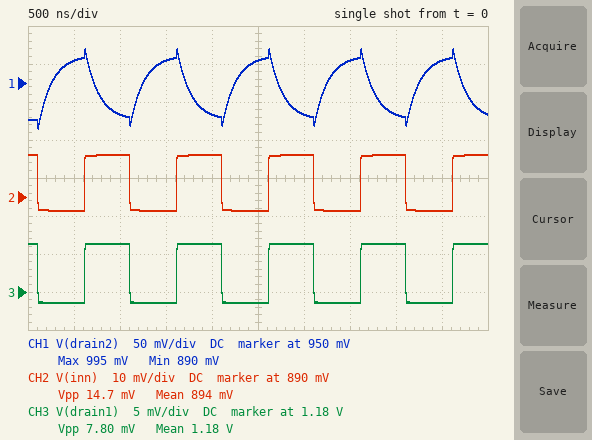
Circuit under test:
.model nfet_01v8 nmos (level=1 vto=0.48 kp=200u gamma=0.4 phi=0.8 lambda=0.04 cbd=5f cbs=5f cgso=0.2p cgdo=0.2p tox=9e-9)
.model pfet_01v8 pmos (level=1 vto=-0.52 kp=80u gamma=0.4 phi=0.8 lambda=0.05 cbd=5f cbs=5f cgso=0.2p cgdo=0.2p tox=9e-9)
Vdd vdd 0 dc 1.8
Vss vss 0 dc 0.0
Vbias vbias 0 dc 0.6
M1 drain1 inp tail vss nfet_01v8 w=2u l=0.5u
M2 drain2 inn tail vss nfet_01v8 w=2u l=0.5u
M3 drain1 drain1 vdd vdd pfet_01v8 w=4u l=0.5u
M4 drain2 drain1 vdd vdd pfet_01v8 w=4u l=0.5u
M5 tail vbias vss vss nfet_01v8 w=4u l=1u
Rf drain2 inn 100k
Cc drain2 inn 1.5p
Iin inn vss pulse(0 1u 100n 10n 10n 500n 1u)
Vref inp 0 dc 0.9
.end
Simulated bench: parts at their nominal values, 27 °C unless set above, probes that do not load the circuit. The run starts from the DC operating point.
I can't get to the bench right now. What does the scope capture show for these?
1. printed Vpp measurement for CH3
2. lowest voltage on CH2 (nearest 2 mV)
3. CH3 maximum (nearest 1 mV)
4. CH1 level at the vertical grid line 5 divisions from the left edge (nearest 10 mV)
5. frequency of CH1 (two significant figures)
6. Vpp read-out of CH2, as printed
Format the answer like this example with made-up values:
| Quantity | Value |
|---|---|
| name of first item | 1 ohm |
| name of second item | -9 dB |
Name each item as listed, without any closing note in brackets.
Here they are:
| Quantity | Value |
|---|---|
| printed Vpp measurement for CH3 | 7.80 mV |
| lowest voltage on CH2 | 886 mV |
| CH3 maximum | 1.186 V |
| CH1 level at the vertical grid line 5 divisions from the left edge | 980 mV |
| frequency of CH1 | 1.0 MHz |
| Vpp read-out of CH2, as printed | 14.7 mV |
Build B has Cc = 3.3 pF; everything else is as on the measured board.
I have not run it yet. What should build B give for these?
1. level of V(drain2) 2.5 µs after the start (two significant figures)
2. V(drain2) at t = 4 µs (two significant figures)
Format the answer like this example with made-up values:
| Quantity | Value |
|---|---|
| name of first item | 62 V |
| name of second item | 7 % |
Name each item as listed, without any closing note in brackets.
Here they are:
| Quantity | Value |
|---|---|
| level of V(drain2) 2.5 µs after the start | 960 mV |
| V(drain2) at t = 4 µs | 930 mV |
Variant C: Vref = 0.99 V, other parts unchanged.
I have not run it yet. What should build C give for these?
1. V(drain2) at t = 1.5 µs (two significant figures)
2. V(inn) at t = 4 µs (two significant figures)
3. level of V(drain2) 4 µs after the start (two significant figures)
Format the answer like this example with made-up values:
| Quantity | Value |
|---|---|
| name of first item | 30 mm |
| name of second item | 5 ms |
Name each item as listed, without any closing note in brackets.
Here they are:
| Quantity | Value |
|---|---|
| V(drain2) at t = 1.5 µs | 1.1 V |
| V(inn) at t = 4 µs | 990 mV |
| level of V(drain2) 4 µs after the start | 1.0 V |
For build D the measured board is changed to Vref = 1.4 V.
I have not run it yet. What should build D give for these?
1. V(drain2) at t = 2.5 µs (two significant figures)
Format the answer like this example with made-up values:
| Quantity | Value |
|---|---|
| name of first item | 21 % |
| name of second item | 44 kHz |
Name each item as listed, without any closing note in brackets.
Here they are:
| Quantity | Value |
|---|---|
| V(drain2) at t = 2.5 µs | 1.5 V |
